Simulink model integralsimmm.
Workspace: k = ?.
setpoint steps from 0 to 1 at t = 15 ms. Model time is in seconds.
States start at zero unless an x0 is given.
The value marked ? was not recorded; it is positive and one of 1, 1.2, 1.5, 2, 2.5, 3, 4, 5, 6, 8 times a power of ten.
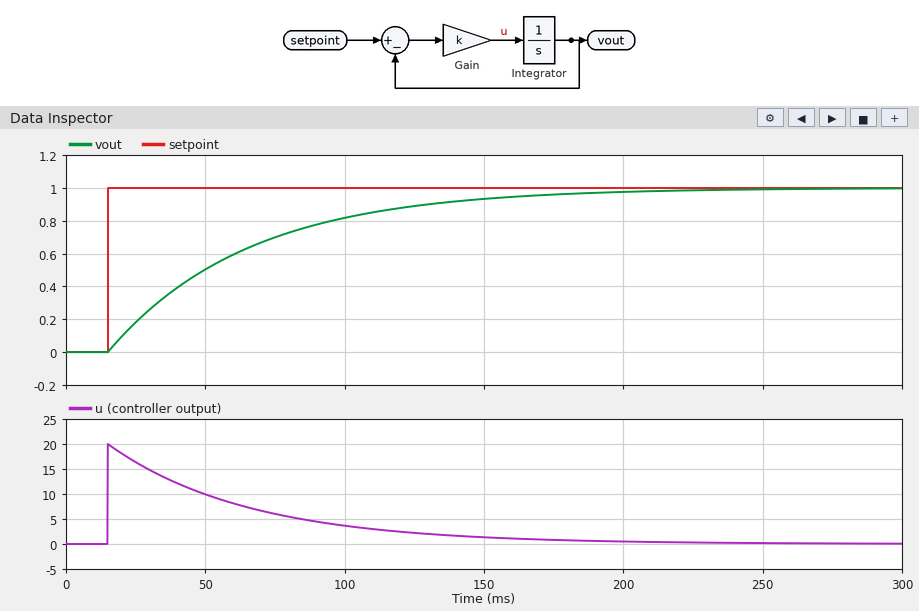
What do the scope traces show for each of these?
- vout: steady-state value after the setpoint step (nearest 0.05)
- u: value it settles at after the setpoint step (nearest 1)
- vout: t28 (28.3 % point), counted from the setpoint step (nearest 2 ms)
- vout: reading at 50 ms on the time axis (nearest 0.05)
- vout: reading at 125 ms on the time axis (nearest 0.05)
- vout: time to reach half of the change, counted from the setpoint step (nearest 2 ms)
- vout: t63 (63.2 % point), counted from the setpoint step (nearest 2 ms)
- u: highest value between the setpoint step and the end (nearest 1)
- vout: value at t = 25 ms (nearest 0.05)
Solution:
1.00
0
16 ms
0.50
0.90
34 ms
50 ms
20
0.20
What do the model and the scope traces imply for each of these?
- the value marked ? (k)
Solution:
20
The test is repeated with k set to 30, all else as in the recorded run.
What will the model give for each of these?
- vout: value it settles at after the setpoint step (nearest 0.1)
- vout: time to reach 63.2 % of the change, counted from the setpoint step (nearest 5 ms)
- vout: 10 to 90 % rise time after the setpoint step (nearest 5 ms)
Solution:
1.0
35 ms
75 ms
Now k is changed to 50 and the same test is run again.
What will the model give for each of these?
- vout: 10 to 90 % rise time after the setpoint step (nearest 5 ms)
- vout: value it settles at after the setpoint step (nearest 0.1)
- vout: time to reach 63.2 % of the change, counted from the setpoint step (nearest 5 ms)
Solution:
45 ms
1.0
20 ms
